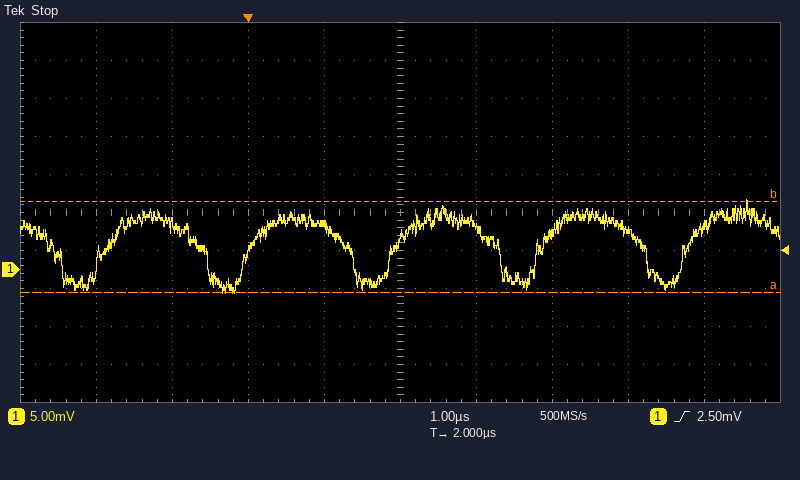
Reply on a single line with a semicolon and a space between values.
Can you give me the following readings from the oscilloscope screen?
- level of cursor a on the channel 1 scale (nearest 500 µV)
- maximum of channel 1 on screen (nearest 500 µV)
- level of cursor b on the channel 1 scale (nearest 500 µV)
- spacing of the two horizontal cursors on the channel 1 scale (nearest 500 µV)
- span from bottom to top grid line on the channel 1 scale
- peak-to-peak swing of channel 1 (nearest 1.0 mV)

-3.0 mV; 9.0 mV; 9.0 mV; 12.0 mV; 50 mV; 12.0 mV
